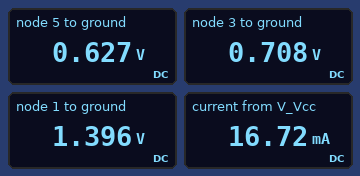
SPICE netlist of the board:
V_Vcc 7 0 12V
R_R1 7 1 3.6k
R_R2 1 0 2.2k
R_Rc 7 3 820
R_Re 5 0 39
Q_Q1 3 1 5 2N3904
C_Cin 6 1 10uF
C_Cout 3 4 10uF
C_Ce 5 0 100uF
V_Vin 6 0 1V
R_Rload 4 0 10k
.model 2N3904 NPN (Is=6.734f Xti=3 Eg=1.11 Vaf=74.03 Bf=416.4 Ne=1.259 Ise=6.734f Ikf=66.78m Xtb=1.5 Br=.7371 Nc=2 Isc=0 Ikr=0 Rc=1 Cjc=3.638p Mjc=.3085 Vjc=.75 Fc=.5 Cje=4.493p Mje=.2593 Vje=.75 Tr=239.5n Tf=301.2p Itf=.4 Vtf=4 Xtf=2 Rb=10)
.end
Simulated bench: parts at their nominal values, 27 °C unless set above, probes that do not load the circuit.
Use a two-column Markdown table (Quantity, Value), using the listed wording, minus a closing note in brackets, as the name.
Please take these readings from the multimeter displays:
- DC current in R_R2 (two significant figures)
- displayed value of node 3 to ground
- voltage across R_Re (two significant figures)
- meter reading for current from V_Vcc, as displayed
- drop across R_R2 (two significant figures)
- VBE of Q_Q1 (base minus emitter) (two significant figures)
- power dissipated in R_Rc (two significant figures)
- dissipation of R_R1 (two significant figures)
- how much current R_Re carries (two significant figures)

| Quantity | Value |
|---|---|
| DC current in R_R2 | 630 µA |
| displayed value of node 3 to ground | 0.708 V |
| voltage across R_Re | 630 mV |
| meter reading for current from V_Vcc, as displayed | 16.72 mA |
| drop across R_R2 | 1.4 V |
| VBE of Q_Q1 (base minus emitter) | 770 mV |
| power dissipated in R_Rc | 160 mW |
| dissipation of R_R1 | 31 mW |
| how much current R_Re carries | 16 mA |
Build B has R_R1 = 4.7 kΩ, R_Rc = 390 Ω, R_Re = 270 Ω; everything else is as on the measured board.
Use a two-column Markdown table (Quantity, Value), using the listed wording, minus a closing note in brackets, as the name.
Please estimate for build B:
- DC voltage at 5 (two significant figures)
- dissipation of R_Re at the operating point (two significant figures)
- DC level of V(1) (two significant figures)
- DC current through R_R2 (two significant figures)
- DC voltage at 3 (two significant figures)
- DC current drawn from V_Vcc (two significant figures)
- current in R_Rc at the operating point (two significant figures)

| Quantity | Value |
|---|---|
| DC voltage at 5 | 3.0 V |
| dissipation of R_Re at the operating point | 33 mW |
| DC level of V(1) | 3.7 V |
| DC current through R_R2 | 1.7 mA |
| DC voltage at 3 | 7.7 V |
| DC current drawn from V_Vcc | 13 mA |
| current in R_Rc at the operating point | 11 mA |
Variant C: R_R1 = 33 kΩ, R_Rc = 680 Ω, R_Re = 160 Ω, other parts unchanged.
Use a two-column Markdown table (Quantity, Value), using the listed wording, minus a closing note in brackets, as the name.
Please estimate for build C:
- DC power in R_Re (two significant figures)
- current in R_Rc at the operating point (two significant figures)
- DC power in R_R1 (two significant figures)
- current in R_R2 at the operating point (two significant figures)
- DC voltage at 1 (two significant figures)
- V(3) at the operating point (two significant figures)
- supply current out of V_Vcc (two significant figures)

| Quantity | Value |
|---|---|
| DC power in R_Re | 55 µW |
| current in R_Rc at the operating point | 580 µA |
| DC power in R_R1 | 3.8 mW |
| current in R_R2 at the operating point | 340 µA |
| DC voltage at 1 | 740 mV |
| V(3) at the operating point | 12 V |
| supply current out of V_Vcc | 920 µA |
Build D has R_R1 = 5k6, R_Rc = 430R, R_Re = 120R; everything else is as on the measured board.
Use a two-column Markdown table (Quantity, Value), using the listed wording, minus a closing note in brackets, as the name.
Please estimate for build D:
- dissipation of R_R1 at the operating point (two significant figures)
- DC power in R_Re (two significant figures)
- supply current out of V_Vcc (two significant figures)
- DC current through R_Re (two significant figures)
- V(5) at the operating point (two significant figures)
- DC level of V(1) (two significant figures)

| Quantity | Value |
|---|---|
| dissipation of R_R1 at the operating point | 14 mW |
| DC power in R_Re | 49 mW |
| supply current out of V_Vcc | 22 mA |
| DC current through R_Re | 20 mA |
| V(5) at the operating point | 2.4 V |
| DC level of V(1) | 3.2 V |
